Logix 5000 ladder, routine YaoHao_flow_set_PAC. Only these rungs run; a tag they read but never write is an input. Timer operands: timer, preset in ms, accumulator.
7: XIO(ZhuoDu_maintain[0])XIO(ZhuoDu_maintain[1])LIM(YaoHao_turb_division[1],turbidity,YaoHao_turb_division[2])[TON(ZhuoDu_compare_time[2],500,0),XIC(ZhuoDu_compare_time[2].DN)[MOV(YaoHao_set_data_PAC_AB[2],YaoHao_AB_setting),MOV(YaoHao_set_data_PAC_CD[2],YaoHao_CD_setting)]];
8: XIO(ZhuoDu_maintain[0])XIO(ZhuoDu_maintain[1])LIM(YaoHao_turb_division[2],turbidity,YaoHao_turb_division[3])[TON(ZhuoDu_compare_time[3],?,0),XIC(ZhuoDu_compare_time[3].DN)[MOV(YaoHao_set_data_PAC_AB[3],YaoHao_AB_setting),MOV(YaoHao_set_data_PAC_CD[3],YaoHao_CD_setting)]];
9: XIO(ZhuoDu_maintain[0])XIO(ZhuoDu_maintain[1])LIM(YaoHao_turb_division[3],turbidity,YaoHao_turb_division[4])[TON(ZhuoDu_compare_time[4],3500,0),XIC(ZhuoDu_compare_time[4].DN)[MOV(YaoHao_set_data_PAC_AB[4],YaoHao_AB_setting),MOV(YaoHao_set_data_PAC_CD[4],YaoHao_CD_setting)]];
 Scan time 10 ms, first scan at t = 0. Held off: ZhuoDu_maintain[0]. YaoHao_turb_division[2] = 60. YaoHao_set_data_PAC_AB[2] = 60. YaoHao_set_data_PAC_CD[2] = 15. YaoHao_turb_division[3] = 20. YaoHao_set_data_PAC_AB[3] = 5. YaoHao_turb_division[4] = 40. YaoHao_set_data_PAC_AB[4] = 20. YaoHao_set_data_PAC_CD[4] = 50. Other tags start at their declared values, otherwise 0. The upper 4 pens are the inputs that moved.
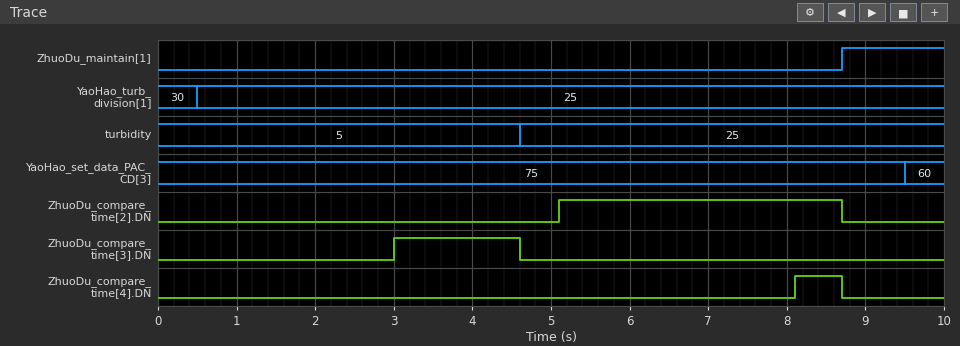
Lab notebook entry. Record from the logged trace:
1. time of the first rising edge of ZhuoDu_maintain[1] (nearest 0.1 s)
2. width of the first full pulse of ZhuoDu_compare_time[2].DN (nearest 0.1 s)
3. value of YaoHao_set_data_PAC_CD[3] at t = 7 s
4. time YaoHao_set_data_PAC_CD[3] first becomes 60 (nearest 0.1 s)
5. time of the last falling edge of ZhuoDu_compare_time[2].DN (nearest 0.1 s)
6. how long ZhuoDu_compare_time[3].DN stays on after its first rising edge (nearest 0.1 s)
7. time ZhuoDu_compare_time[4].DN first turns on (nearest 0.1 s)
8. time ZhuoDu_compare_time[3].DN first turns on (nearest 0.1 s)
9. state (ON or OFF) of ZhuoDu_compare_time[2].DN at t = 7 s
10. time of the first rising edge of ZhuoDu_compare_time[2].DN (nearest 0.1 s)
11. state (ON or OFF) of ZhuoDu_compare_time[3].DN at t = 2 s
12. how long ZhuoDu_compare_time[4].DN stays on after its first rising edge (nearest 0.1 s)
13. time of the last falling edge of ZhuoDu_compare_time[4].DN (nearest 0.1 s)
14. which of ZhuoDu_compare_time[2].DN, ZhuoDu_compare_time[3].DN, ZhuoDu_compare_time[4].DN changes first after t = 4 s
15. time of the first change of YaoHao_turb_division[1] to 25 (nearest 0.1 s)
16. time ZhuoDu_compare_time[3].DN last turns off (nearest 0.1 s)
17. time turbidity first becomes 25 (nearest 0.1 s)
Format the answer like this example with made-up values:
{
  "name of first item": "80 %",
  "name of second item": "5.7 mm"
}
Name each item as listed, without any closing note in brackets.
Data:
{
  "time of the first rising edge of ZhuoDu_maintain[1]": "8.7 s",
  "width of the first full pulse of ZhuoDu_compare_time[2].DN": "3.6 s",
  "value of YaoHao_set_data_PAC_CD[3] at t = 7 s": "75",
  "time YaoHao_set_data_PAC_CD[3] first becomes 60": "9.5 s",
  "time of the last falling edge of ZhuoDu_compare_time[2].DN": "8.7 s",
  "how long ZhuoDu_compare_time[3].DN stays on after its first rising edge": "1.6 s",
  "time ZhuoDu_compare_time[4].DN first turns on": "8.1 s",
  "time ZhuoDu_compare_time[3].DN first turns on": "3.0 s",
  "state (ON or OFF) of ZhuoDu_compare_time[2].DN at t = 7 s": "ON",
  "time of the first rising edge of ZhuoDu_compare_time[2].DN": "5.1 s",
  "state (ON or OFF) of ZhuoDu_compare_time[3].DN at t = 2 s": "OFF",
  "how long ZhuoDu_compare_time[4].DN stays on after its first rising edge": "0.6 s",
  "time of the last falling edge of ZhuoDu_compare_time[4].DN": "8.7 s",
  "which of ZhuoDu_compare_time[2].DN, ZhuoDu_compare_time[3].DN, ZhuoDu_compare_time[4].DN changes first after t = 4 s": "ZhuoDu_compare_time[3].DN",
  "time of the first change of YaoHao_turb_division[1] to 25": "0.5 s",
  "time ZhuoDu_compare_time[3].DN last turns off": "4.6 s",
  "time turbidity first becomes 25": "4.6 s"
}
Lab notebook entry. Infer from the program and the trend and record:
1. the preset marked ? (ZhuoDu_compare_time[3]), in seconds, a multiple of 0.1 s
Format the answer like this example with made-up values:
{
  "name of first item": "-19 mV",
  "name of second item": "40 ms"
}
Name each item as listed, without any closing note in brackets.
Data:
{
  "the preset marked ? (ZhuoDu_compare_time[3]), in seconds, a multiple of 0.1 s": "3.0 s"
}
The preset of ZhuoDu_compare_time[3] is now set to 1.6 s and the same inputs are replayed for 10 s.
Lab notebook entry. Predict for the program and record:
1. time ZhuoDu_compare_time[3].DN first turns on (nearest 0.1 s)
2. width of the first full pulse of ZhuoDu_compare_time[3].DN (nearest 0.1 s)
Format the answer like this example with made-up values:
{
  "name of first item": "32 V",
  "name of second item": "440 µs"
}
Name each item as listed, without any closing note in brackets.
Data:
{
  "time ZhuoDu_compare_time[3].DN first turns on": "1.6 s",
  "width of the first full pulse of ZhuoDu_compare_time[3].DN": "3.0 s"
}
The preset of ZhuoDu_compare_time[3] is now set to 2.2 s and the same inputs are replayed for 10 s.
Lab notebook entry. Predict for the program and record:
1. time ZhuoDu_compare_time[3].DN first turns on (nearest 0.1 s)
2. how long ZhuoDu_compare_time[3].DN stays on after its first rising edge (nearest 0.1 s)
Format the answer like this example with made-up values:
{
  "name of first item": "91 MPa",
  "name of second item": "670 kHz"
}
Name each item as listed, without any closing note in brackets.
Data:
{
  "time ZhuoDu_compare_time[3].DN first turns on": "2.2 s",
  "how long ZhuoDu_compare_time[3].DN stays on after its first rising edge": "2.4 s"
}
